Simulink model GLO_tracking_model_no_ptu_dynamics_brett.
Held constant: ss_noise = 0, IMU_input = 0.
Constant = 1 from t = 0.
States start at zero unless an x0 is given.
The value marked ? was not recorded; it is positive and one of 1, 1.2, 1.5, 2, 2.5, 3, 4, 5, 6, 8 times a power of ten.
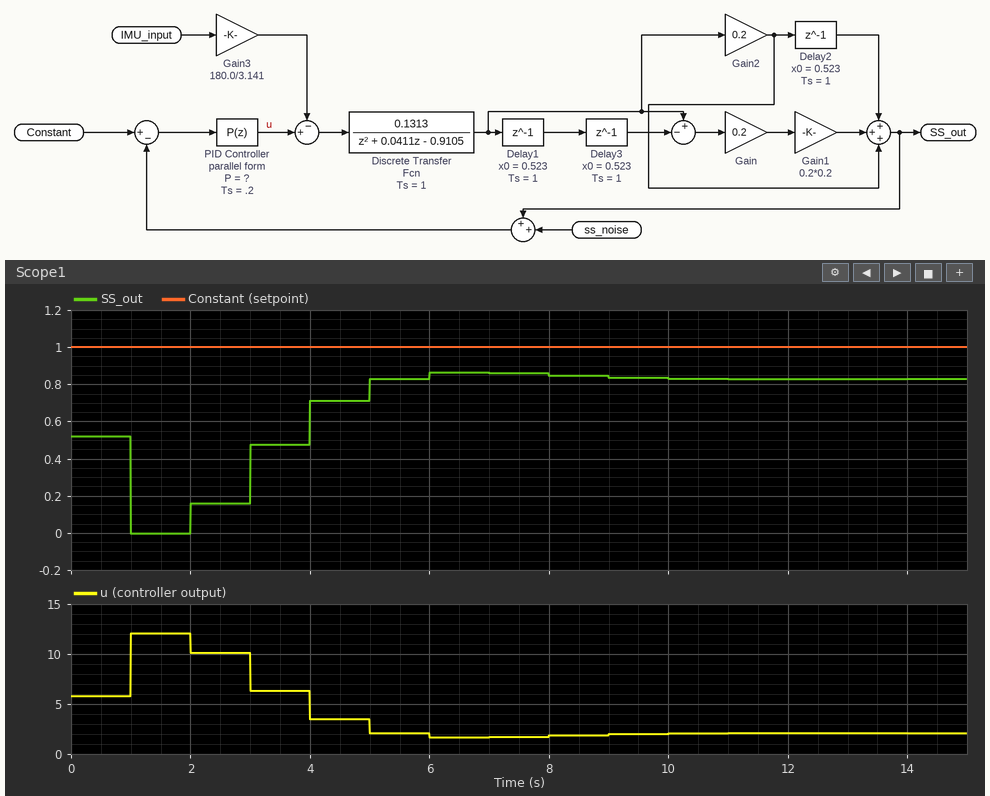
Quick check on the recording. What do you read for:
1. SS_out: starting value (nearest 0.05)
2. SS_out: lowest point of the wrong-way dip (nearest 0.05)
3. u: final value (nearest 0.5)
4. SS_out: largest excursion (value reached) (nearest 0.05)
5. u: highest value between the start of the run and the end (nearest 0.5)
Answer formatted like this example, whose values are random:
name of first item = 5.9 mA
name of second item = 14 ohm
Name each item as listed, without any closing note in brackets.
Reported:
SS_out: starting value = 0.50
SS_out: lowest point of the wrong-way dip = 0.00
u: final value = 2.0
SS_out: largest excursion (value reached) = 0.85
u: highest value between the start of the run and the end = 12.0
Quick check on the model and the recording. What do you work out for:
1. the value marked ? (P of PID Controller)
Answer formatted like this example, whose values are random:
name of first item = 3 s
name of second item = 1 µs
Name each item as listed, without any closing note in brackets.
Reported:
the value marked ? = 12
